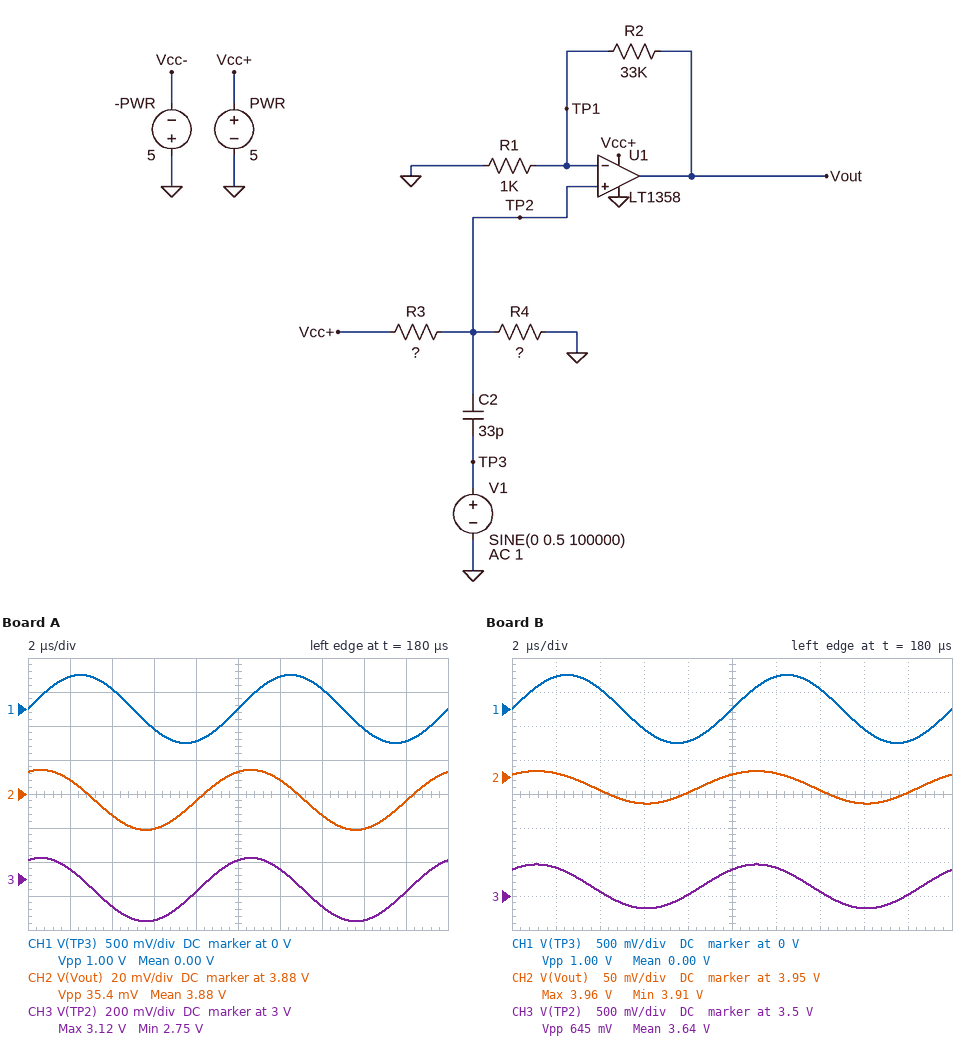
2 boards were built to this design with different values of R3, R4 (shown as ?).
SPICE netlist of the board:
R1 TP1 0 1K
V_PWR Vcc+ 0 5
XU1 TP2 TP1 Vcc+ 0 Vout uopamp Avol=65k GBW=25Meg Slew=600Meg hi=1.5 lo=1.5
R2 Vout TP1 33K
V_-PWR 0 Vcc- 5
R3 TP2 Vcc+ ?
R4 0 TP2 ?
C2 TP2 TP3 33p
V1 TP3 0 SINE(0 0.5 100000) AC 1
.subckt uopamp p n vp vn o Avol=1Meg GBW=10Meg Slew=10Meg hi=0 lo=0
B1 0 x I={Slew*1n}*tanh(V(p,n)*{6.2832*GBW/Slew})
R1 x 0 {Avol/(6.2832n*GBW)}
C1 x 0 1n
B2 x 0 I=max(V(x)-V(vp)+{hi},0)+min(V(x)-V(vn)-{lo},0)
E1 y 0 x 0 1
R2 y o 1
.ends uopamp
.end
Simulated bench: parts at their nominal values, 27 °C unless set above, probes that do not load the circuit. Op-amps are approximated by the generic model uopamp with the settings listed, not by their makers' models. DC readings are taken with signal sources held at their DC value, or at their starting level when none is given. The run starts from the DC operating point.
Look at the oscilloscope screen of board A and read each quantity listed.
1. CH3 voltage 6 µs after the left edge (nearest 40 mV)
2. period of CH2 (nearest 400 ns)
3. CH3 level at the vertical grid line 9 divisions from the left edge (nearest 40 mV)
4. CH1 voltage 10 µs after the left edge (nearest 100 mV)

2.76 V
10.0 µs
2.92 V
0 V
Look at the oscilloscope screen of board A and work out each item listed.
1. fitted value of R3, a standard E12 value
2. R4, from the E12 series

33 kΩ
47 kΩ
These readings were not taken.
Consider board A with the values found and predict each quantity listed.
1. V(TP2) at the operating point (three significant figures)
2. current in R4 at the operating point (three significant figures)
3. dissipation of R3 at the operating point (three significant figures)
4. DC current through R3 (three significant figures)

2.94 V
62.5 µA
129 µW
62.5 µA
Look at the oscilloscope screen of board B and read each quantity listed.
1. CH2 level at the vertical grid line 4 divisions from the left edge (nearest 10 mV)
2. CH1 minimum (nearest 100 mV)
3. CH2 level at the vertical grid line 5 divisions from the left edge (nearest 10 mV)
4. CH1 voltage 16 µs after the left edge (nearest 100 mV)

3.93 V
-500 mV
3.95 V
-300 mV
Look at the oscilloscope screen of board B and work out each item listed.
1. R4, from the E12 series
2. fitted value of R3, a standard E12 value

150 kΩ
56 kΩ
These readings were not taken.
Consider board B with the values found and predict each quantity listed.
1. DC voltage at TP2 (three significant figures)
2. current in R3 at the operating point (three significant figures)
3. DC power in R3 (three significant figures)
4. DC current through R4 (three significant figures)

3.64 V
24.3 µA
33.0 µW
24.3 µA
